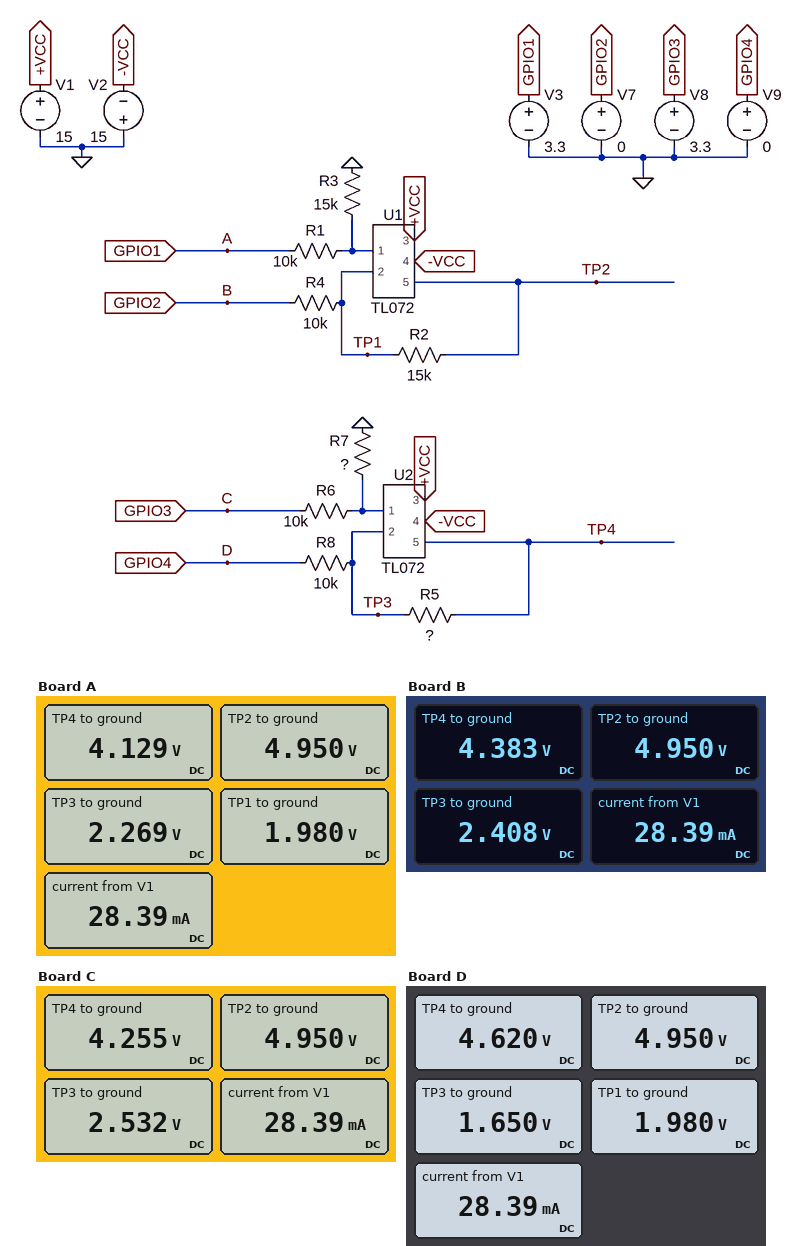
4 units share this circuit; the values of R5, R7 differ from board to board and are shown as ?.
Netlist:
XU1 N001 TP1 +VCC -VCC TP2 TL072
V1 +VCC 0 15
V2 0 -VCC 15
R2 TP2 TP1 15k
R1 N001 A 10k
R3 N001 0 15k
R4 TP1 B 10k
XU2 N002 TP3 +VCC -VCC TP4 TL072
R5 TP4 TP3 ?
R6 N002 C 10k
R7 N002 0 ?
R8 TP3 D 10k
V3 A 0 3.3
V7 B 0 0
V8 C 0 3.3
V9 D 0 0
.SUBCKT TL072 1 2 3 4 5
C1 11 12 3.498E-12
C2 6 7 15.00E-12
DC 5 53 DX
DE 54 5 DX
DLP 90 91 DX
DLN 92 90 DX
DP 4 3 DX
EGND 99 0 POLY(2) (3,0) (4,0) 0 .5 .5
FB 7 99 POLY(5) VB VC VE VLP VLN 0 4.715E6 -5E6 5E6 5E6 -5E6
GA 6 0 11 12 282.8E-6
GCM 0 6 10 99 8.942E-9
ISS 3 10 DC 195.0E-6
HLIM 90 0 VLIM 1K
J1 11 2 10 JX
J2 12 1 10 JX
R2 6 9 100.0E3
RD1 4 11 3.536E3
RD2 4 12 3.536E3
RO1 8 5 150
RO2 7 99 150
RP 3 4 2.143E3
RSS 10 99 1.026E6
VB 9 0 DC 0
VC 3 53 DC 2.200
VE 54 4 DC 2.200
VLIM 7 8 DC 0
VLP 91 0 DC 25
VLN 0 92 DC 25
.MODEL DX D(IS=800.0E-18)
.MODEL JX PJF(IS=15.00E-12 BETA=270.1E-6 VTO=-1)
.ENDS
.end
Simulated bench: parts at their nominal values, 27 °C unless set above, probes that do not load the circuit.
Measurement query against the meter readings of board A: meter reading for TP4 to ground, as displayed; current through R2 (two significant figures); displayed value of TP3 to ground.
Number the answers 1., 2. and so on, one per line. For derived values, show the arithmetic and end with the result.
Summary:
1. 4.129 V
2. (4.95 V - 1.98 V) / 15 kΩ = 200 µA
3. 2.269 V
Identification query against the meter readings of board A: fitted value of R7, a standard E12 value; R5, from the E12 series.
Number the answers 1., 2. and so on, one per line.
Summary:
1. 22 kΩ
2. 8.2 kΩ
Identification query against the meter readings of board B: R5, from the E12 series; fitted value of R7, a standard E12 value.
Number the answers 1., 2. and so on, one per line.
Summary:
1. 8.2 kΩ
2. 27 kΩ
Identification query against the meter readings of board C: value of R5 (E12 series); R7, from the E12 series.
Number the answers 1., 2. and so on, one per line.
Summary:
1. 6.8 kΩ
2. 33 kΩ
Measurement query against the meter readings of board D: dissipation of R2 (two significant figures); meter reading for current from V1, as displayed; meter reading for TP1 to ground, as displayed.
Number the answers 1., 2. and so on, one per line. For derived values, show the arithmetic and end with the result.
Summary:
1. (4.95 V - 1.98 V)^2 / 15 kΩ = 590 µW
2. 28.39 mA
3. 1.980 V
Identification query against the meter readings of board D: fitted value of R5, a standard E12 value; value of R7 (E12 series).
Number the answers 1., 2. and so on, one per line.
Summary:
1. 18 kΩ
2. 10 kΩ
